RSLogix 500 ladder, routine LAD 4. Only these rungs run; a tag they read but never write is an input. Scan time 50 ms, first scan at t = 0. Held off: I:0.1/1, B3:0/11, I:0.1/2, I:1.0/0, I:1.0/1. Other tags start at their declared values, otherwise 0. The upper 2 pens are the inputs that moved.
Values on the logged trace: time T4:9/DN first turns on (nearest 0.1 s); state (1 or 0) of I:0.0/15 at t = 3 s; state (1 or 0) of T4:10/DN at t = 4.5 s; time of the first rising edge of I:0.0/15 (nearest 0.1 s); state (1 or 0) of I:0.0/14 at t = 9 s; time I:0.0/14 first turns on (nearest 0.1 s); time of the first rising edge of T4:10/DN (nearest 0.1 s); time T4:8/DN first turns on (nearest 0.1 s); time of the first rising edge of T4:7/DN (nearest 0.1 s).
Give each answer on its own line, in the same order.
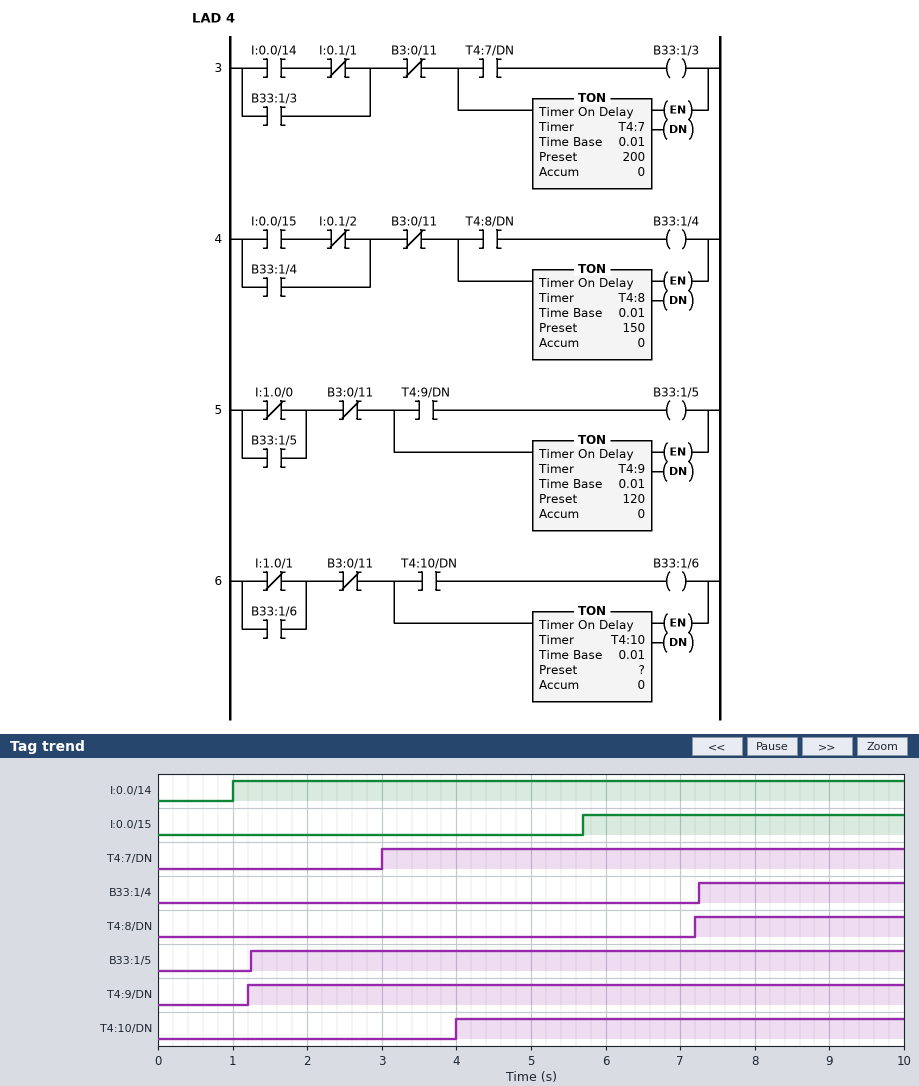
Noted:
1.2 s
0
1
5.7 s
1
1.0 s
4.0 s
7.2 s
3.0 s
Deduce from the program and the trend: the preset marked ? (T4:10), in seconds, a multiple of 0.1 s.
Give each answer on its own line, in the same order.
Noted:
4.0 s
